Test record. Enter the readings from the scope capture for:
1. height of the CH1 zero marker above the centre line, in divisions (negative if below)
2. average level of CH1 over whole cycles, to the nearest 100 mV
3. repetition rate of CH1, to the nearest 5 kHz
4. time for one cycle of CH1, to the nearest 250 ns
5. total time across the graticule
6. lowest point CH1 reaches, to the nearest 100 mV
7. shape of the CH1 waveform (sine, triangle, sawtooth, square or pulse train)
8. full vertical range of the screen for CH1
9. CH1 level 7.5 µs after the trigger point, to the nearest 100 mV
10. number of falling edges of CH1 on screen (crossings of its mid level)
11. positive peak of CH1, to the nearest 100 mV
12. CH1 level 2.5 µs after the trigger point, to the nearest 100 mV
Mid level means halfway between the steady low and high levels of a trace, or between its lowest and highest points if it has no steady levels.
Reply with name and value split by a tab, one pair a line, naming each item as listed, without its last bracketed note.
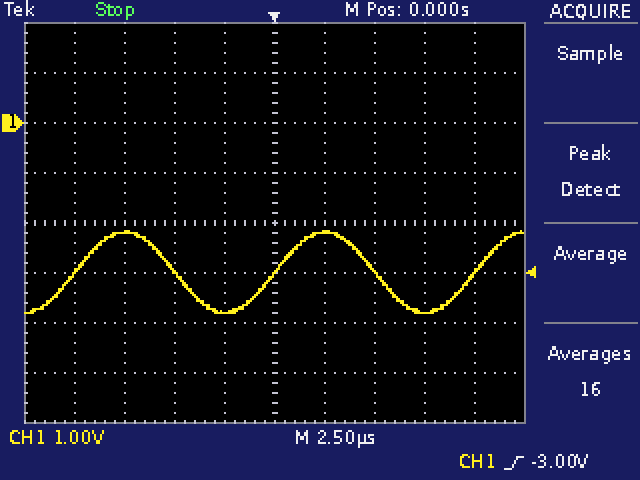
height of the CH1 zero marker above the centre line, in divisions	+2.0 div
average level of CH1 over whole cycles, to the nearest 100 mV	-3.0 V
repetition rate of CH1, to the nearest 5 kHz	100 kHz
time for one cycle of CH1, to the nearest 250 ns	10.00 µs
total time across the graticule	25 µs
lowest point CH1 reaches, to the nearest 100 mV	-3.8 V
shape of the CH1 waveform	sine
full vertical range of the screen for CH1	8 V
CH1 level 7.5 µs after the trigger point, to the nearest 100 mV	-3.8 V
number of falling edges of CH1 on screen	2
positive peak of CH1, to the nearest 100 mV	-2.2 V
CH1 level 2.5 µs after the trigger point, to the nearest 100 mV	-2.2 V
